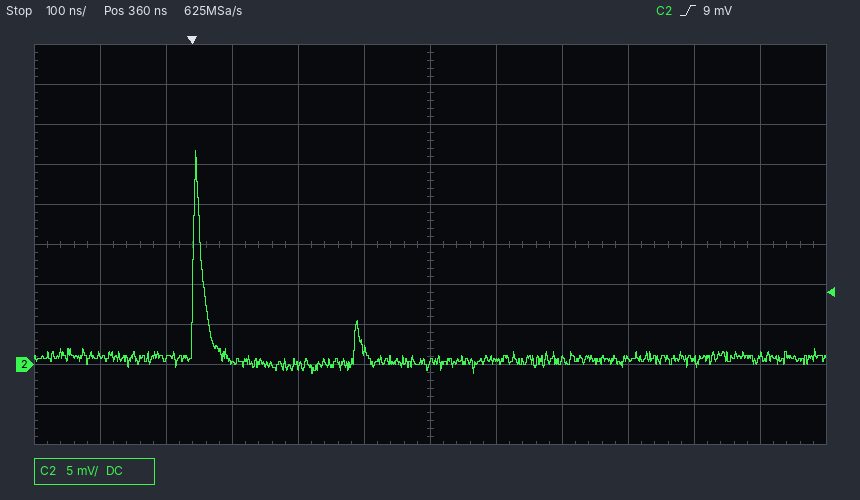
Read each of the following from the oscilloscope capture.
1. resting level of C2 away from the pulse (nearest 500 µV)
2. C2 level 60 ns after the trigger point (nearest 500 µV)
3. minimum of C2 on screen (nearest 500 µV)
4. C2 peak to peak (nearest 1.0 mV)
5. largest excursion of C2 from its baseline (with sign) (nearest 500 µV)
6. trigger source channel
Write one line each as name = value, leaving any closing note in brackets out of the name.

resting level of C2 away from the pulse = 500 µV
C2 level 60 ns after the trigger point = 500 µV
minimum of C2 on screen = -1.0 mV
C2 peak to peak = 28.0 mV
largest excursion of C2 from its baseline (with sign) = +26.0 mV
trigger source channel = C2
